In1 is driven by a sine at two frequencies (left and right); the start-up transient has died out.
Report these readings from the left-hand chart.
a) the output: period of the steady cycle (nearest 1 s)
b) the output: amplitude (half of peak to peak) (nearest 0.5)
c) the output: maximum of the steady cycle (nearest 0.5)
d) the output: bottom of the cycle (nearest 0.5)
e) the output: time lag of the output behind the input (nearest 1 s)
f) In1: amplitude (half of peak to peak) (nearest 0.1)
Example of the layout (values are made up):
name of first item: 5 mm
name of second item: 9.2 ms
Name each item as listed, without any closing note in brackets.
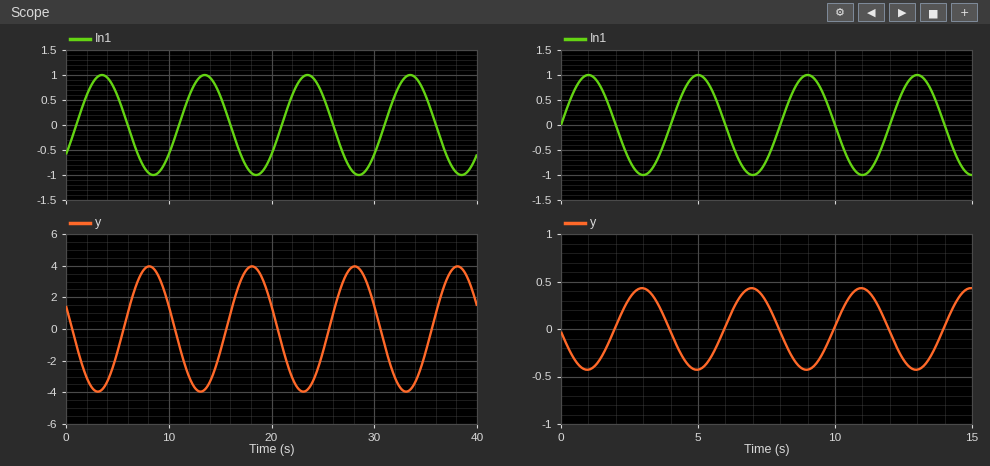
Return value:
the output: period of the steady cycle: 10 s
the output: amplitude (half of peak to peak): 4.0
the output: maximum of the steady cycle: 4.0
the output: bottom of the cycle: -4.0
the output: time lag of the output behind the input: 5 s
In1: amplitude (half of peak to peak): 1.0
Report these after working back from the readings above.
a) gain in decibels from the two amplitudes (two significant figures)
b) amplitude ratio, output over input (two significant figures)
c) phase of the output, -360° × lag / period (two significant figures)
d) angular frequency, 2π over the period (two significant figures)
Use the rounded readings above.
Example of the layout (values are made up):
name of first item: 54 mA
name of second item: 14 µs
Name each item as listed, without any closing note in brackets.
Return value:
gain in decibels from the two amplitudes: 12 dB
amplitude ratio, output over input: 4.0
phase of the output, -360° × lag / period: -180°
angular frequency, 2π over the period: 0.63 rad/s
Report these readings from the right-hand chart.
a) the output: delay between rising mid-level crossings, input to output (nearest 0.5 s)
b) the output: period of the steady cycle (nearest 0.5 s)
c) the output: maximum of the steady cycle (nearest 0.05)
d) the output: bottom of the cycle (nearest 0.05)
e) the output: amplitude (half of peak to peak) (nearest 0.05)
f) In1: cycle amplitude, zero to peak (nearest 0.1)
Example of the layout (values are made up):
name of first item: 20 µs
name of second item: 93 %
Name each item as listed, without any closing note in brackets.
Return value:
the output: delay between rising mid-level crossings, input to output: 2.0 s
the output: period of the steady cycle: 4.0 s
the output: maximum of the steady cycle: 0.45
the output: bottom of the cycle: -0.45
the output: amplitude (half of peak to peak): 0.45
In1: cycle amplitude, zero to peak: 1.0
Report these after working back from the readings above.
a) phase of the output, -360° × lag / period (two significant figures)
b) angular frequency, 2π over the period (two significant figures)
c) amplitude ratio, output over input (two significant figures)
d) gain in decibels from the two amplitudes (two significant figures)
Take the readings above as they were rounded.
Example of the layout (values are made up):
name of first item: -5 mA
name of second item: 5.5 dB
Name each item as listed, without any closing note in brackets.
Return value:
phase of the output, -360° × lag / period: -180°
angular frequency, 2π over the period: 1.6 rad/s
amplitude ratio, output over input: 0.45
gain in decibels from the two amplitudes: -6.9 dB
